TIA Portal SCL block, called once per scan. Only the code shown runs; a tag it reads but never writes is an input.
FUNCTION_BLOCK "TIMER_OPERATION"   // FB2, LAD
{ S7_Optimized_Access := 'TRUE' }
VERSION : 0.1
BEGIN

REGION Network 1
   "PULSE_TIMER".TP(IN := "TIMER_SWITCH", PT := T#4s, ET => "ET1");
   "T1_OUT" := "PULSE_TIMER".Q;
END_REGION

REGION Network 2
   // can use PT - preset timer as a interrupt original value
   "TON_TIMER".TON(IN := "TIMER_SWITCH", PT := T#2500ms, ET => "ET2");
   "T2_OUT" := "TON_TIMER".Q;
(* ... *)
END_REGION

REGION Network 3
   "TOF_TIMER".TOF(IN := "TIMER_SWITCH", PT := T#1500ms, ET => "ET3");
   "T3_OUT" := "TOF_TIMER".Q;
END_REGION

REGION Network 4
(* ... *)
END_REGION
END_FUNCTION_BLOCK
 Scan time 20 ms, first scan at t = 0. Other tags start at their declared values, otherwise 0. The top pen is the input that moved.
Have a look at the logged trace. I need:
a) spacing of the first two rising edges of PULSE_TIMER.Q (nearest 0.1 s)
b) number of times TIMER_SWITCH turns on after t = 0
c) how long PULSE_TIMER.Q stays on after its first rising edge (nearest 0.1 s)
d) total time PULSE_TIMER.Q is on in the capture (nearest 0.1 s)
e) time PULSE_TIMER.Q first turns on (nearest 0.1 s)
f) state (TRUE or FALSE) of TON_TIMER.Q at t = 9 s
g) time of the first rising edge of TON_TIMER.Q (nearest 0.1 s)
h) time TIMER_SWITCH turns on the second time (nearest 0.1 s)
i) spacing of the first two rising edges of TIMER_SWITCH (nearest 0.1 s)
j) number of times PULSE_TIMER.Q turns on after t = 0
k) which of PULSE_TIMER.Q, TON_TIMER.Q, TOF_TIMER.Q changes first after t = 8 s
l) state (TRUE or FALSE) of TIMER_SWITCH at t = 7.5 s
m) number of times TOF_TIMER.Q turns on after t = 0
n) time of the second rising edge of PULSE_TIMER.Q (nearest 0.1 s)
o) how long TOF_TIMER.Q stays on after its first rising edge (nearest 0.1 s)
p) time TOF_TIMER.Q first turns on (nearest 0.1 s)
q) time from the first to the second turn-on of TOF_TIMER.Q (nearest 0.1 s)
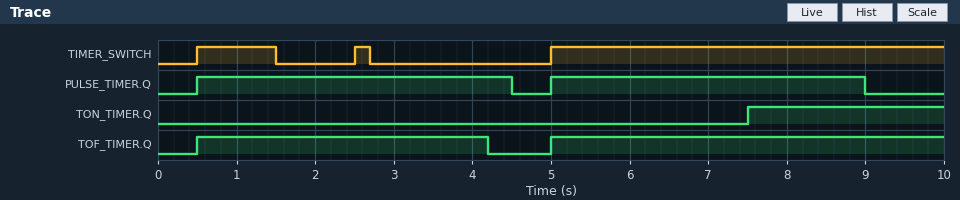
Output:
4.5 s
3
4.0 s
8.0 s
0.5 s
TRUE
7.5 s
2.5 s
2.0 s
2
PULSE_TIMER.Q
TRUE
2
5.0 s
3.7 s
0.5 s
4.5 s
